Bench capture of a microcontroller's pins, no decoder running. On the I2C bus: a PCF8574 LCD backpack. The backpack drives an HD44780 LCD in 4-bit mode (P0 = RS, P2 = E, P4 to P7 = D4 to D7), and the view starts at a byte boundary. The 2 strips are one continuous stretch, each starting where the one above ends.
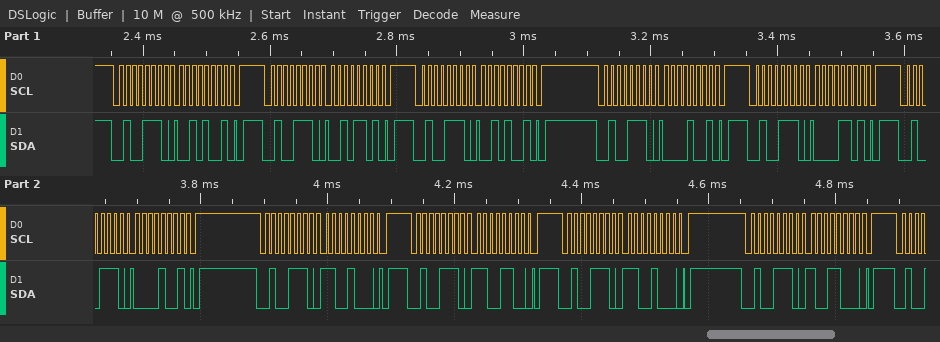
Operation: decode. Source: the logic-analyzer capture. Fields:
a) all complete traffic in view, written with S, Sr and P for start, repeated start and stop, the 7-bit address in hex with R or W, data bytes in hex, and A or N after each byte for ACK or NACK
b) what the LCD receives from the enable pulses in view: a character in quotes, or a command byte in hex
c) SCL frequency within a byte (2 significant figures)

S 27W A 29 A P S 27W A 2D A P S 27W A 29 A P S 27W A 09 A P S 27W A 0D A P S 27W A 09 A P S 27W A C8 A P S 27W A CC A P S 27W A C8 A P S 27W A 98 A P
' '
100 kHz
